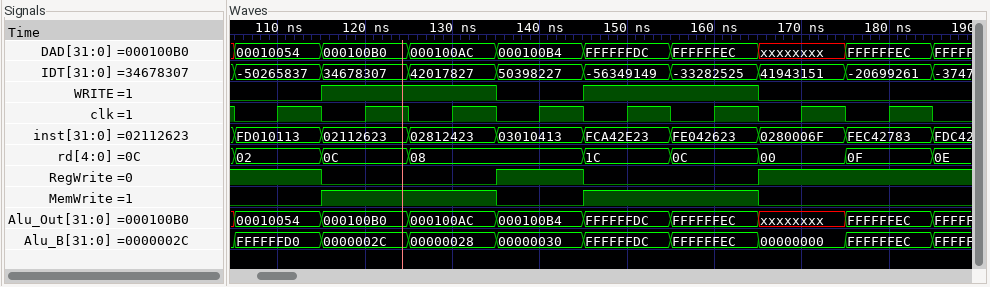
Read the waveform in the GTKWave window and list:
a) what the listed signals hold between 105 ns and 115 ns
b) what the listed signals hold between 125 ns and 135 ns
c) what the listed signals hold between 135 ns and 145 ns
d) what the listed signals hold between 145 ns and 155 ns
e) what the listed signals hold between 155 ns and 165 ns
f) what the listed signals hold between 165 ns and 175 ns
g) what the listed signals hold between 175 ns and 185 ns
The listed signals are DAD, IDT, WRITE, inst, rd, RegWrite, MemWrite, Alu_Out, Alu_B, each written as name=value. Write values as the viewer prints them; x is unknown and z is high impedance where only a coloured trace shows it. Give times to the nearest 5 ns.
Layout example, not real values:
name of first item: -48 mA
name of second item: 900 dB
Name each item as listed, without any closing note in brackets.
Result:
what the listed signals hold between 105 ns and 115 ns: DAD=00010054, IDT=-50265837, WRITE=0, inst=FD010113, rd=02, RegWrite=1, MemWrite=0, Alu_Out=00010054, Alu_B=FFFFFFD0
what the listed signals hold between 125 ns and 135 ns: DAD=000100AC, IDT=42017827, WRITE=1, inst=02812423, rd=08, RegWrite=0, MemWrite=1, Alu_Out=000100AC, Alu_B=00000028
what the listed signals hold between 135 ns and 145 ns: DAD=000100B4, IDT=50398227, WRITE=0, inst=03010413, rd=08, RegWrite=1, MemWrite=0, Alu_Out=000100B4, Alu_B=00000030
what the listed signals hold between 145 ns and 155 ns: DAD=FFFFFFDC, IDT=-56349149, WRITE=1, inst=FCA42E23, rd=1C, RegWrite=0, MemWrite=1, Alu_Out=FFFFFFDC, Alu_B=FFFFFFDC
what the listed signals hold between 155 ns and 165 ns: DAD=FFFFFFEC, IDT=-33282525, WRITE=1, inst=FE042623, rd=0C, RegWrite=0, MemWrite=1, Alu_Out=FFFFFFEC, Alu_B=FFFFFFEC
what the listed signals hold between 165 ns and 175 ns: DAD=xxxxxxxx, IDT=41943151, WRITE=0, inst=0280006F, rd=00, RegWrite=1, MemWrite=0, Alu_Out=xxxxxxxx, Alu_B=00000000
what the listed signals hold between 175 ns and 185 ns: DAD=FFFFFFEC, IDT=-20699261, WRITE=0, inst=FEC42783, rd=0F, RegWrite=1, MemWrite=0, Alu_Out=FFFFFFEC, Alu_B=FFFFFFEC
